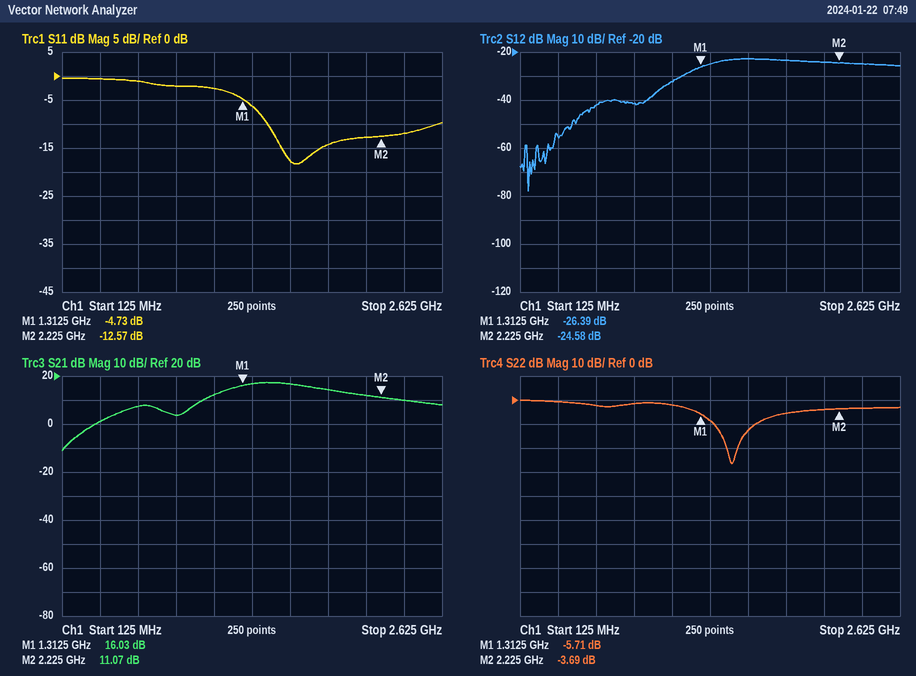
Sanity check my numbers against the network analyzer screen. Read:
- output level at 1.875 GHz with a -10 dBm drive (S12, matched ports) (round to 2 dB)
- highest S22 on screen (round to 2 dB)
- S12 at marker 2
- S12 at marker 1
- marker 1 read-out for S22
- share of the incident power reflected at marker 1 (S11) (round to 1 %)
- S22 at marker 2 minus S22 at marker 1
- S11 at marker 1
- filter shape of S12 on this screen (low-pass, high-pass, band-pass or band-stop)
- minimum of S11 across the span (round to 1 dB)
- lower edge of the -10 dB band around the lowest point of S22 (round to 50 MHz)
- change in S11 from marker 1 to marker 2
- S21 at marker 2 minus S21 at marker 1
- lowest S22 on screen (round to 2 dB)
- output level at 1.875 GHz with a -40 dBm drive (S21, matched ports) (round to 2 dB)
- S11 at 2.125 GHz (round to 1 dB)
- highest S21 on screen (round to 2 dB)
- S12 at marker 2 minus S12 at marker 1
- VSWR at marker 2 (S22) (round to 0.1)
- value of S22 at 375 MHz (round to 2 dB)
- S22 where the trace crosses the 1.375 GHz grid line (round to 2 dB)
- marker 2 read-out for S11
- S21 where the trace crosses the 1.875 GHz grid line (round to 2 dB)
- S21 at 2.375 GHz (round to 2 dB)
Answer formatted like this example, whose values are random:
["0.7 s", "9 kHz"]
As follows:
["-34 dBm", "0 dB", "-24.58 dB", "-26.39 dB", "-5.71 dB", "34 %", "2.02 dB", "-4.73 dB", "high-pass", "-18 dB", "1.40 GHz", "-7.84 dB", "-4.96 dB", "-26 dB", "-26 dBm", "-13 dB", "18 dB", "1.81 dB", "4.8", "0 dB", "-8 dB", "-12.57 dB", "14 dB", "10 dB"]
